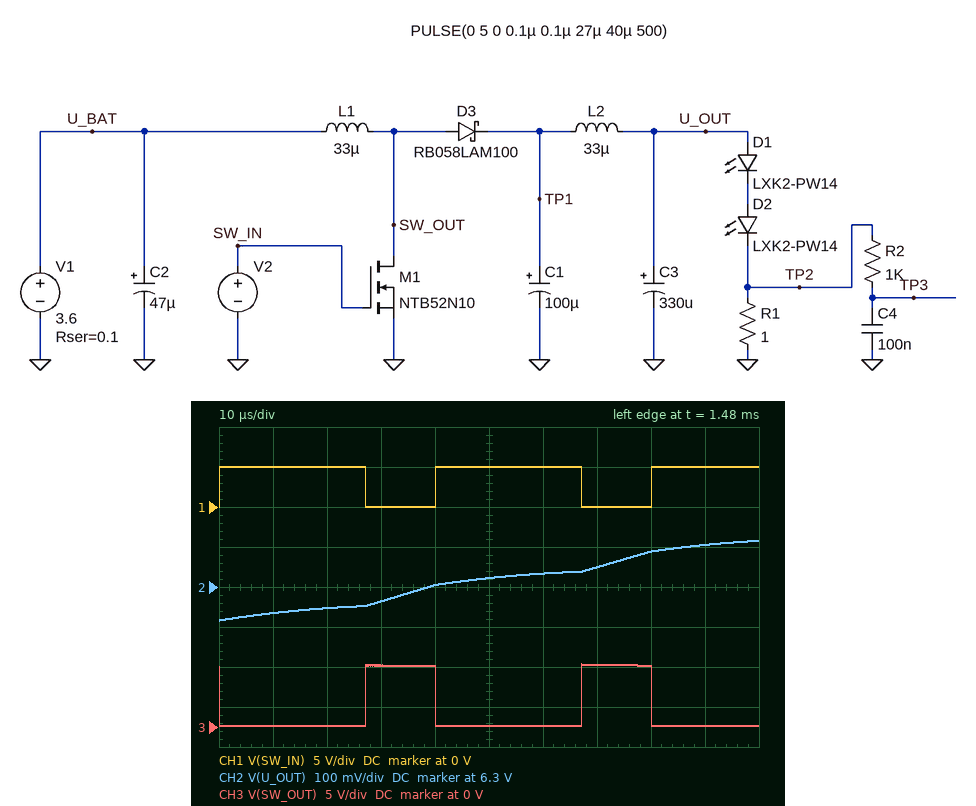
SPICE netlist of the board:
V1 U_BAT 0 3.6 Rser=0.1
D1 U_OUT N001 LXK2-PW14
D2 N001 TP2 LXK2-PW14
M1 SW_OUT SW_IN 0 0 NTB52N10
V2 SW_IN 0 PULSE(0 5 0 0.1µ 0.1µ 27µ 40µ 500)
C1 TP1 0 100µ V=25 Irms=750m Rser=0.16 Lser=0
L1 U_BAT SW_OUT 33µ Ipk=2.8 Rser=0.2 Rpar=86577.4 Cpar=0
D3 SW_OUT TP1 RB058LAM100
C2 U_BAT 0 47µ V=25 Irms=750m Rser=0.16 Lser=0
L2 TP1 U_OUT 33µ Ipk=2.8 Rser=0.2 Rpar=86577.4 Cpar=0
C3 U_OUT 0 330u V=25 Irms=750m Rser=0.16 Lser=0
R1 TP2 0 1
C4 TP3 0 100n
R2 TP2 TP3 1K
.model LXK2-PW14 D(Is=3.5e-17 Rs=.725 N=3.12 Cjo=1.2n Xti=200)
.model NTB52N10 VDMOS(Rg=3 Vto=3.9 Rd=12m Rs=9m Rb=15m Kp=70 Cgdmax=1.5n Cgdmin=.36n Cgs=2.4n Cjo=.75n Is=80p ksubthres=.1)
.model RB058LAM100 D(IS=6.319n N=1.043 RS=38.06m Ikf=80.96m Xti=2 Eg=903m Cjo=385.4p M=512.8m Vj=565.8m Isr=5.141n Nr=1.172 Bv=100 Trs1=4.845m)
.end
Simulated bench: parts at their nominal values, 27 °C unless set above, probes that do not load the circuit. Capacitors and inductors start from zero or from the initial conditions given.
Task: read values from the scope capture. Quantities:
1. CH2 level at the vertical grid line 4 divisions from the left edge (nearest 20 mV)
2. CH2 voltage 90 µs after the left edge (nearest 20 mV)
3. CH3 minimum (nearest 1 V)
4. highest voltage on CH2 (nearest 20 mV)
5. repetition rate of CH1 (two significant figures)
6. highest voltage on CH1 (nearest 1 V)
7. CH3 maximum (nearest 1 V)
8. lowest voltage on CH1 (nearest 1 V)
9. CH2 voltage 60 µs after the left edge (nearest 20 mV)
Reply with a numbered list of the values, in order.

1. 6.30 V
2. 6.40 V
3. 0 V
4. 6.42 V
5. 25 kHz
6. 5 V
7. 8 V
8. 0 V
9. 6.34 V
